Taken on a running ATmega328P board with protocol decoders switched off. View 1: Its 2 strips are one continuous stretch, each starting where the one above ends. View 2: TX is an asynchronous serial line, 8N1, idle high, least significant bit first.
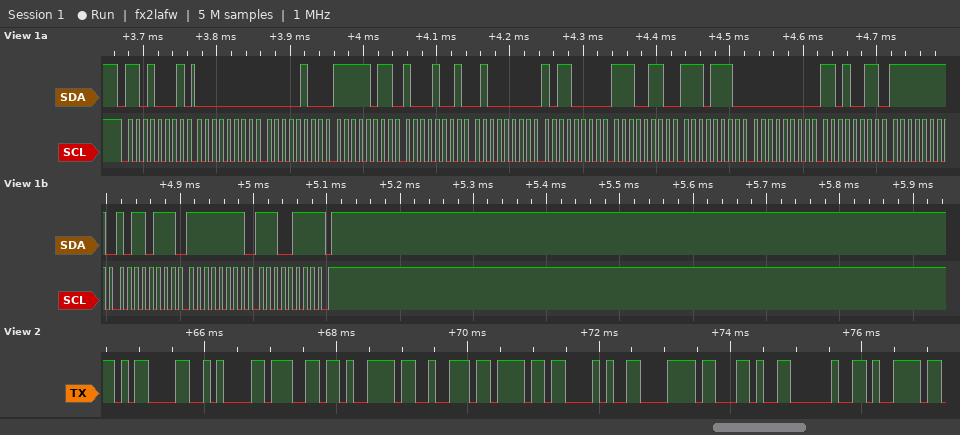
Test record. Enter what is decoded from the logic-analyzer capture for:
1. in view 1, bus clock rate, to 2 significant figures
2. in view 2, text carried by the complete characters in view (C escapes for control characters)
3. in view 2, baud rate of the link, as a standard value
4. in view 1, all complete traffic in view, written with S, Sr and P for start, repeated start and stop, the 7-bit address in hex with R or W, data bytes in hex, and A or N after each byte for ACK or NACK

100 kHz
"\r\ngyro(x, y"
9600 baud
S 68R A 00 A 04 A FB A 89 A 40 A B0 A E6 A EE A 00 A D3 A FF A B7 A FF A E7 N P
